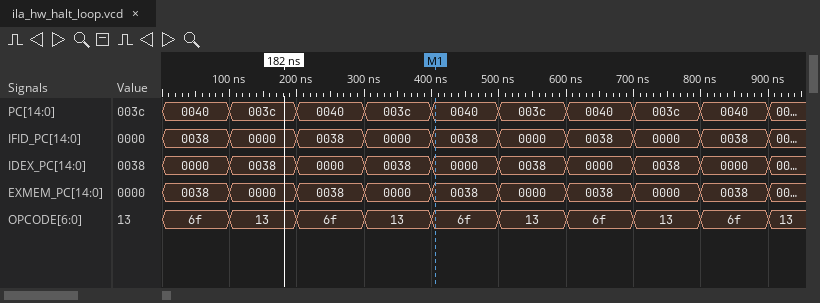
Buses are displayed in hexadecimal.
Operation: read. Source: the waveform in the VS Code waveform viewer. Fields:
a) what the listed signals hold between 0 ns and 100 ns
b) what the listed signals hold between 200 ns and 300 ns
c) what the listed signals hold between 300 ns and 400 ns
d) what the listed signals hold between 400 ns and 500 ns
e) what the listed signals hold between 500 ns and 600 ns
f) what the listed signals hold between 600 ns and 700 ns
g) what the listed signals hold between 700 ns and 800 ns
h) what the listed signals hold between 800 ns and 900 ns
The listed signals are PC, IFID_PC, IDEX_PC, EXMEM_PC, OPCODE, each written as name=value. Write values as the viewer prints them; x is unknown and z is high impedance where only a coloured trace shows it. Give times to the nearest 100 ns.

PC=0040, IFID_PC=0038, IDEX_PC=0000, EXMEM_PC=0038, OPCODE=6f
PC=0040, IFID_PC=0038, IDEX_PC=0000, EXMEM_PC=0038, OPCODE=6f
PC=003c, IFID_PC=0000, IDEX_PC=0038, EXMEM_PC=0000, OPCODE=13
PC=0040, IFID_PC=0038, IDEX_PC=0000, EXMEM_PC=0038, OPCODE=6f
PC=003c, IFID_PC=0000, IDEX_PC=0038, EXMEM_PC=0000, OPCODE=13
PC=0040, IFID_PC=0038, IDEX_PC=0000, EXMEM_PC=0038, OPCODE=6f
PC=003c, IFID_PC=0000, IDEX_PC=0038, EXMEM_PC=0000, OPCODE=13
PC=0040, IFID_PC=0038, IDEX_PC=0000, EXMEM_PC=0038, OPCODE=6f
